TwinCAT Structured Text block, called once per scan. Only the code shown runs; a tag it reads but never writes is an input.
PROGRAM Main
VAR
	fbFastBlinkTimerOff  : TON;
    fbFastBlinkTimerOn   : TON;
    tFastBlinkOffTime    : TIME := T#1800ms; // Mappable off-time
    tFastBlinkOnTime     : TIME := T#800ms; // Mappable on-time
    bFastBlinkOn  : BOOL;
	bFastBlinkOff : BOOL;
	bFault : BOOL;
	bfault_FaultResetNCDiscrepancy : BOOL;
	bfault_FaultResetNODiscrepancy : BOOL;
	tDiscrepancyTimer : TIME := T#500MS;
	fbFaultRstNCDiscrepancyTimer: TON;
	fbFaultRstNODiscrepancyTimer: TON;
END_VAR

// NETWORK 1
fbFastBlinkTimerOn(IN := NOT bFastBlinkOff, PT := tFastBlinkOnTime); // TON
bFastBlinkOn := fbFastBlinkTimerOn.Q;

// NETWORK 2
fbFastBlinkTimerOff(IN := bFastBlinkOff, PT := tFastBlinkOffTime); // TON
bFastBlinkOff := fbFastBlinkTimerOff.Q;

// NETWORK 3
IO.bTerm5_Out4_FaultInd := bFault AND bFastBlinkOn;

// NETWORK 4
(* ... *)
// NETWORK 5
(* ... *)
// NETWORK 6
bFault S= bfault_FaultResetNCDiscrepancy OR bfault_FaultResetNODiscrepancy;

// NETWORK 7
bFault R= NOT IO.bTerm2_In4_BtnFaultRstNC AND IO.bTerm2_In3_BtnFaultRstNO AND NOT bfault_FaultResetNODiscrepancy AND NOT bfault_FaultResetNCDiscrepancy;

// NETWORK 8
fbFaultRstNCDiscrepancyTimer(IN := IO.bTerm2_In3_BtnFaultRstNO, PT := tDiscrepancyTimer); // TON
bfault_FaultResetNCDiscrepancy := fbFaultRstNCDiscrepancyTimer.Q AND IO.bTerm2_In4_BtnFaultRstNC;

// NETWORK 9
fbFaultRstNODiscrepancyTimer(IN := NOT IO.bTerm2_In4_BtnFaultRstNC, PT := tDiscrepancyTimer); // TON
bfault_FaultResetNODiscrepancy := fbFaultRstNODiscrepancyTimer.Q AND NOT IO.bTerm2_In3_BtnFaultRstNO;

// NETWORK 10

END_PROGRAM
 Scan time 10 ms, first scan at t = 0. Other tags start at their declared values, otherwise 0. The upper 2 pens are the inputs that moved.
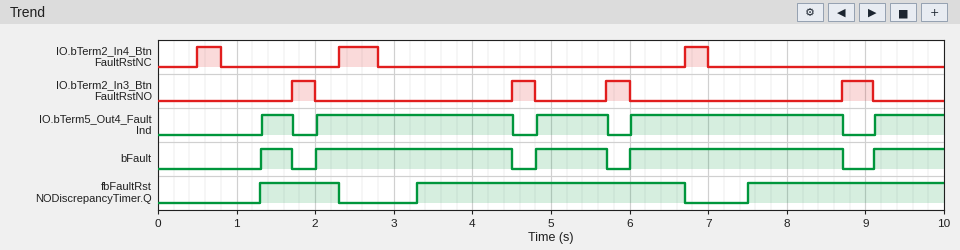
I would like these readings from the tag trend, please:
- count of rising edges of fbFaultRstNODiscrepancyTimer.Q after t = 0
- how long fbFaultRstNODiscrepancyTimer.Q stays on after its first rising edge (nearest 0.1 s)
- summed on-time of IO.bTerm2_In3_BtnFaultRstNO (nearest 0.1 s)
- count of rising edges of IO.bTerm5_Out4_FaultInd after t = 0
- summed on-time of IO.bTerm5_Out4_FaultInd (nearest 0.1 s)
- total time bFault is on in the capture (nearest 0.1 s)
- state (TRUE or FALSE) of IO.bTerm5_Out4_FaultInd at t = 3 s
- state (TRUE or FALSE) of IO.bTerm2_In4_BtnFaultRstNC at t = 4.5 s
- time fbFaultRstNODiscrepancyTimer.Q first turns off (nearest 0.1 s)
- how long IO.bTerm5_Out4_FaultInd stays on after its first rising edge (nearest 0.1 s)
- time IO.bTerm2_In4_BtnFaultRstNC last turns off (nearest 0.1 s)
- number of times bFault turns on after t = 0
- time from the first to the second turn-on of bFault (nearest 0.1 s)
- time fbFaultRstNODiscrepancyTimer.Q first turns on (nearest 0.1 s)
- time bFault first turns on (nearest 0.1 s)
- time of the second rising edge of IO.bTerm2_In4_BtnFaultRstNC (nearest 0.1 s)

3
1.0 s
1.3 s
5
7.4 s
7.4 s
TRUE
FALSE
2.3 s
0.4 s
7.0 s
5
0.7 s
1.3 s
1.3 s
2.3 s
